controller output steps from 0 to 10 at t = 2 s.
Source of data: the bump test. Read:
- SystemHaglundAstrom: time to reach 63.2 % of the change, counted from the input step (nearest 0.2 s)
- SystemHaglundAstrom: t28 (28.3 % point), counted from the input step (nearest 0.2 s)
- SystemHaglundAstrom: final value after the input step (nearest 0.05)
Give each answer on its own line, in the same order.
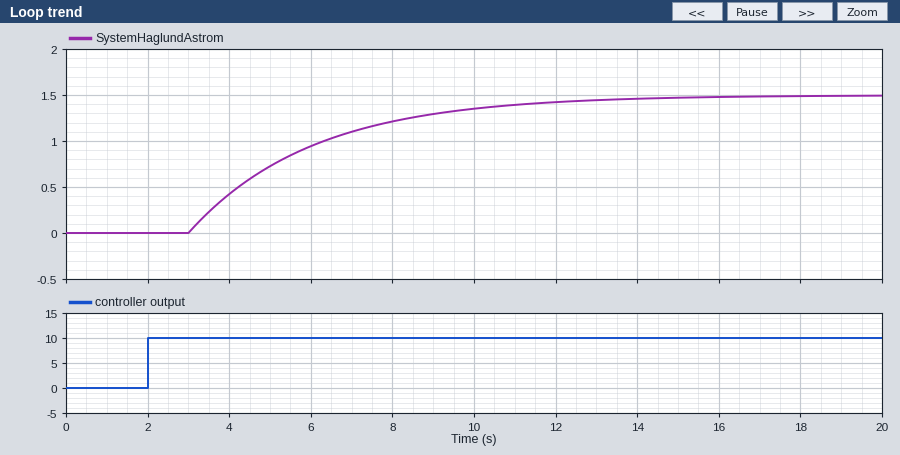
4.0 s
2.0 s
1.50
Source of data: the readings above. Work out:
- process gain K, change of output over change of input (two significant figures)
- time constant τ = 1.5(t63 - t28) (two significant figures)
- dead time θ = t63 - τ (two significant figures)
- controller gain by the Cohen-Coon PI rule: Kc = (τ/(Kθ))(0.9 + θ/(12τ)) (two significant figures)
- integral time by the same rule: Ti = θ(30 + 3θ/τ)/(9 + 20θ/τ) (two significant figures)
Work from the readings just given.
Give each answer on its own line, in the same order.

0.15
3.0 s
1.0 s
19
2.0 s
